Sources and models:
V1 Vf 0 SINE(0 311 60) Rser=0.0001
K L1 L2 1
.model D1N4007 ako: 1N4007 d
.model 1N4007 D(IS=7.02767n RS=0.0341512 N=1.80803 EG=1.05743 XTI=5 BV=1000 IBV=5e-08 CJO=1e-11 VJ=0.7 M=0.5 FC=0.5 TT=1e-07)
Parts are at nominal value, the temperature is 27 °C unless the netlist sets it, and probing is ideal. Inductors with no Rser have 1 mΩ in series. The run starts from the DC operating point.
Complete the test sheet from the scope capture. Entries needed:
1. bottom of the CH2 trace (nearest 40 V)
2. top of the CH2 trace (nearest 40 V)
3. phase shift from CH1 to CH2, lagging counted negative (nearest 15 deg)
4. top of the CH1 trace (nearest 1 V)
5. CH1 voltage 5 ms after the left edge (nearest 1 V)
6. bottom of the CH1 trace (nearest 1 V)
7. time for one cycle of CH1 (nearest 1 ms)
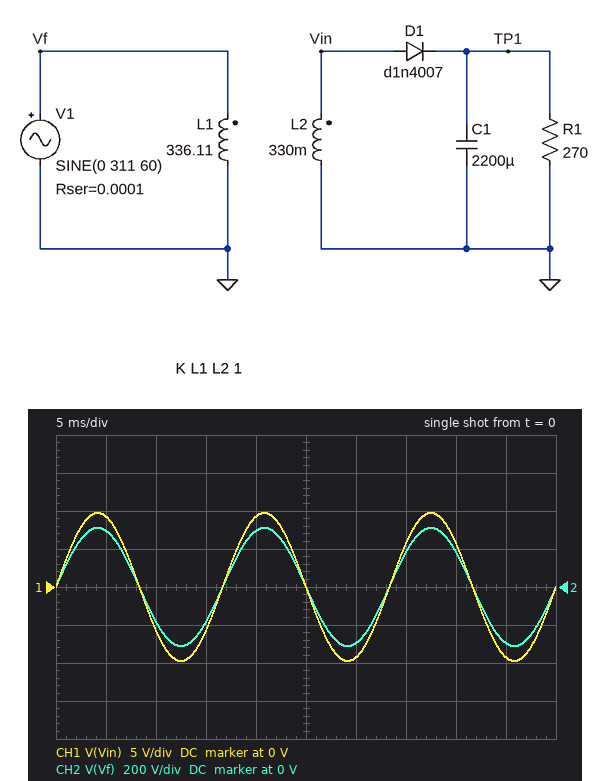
-320 V
320 V
0 deg
10 V
9 V
-10 V
17 ms
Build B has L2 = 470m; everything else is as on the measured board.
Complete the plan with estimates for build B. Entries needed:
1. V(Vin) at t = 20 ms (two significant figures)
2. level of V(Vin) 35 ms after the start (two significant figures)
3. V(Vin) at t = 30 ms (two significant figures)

11 V
6.8 V
-11 V
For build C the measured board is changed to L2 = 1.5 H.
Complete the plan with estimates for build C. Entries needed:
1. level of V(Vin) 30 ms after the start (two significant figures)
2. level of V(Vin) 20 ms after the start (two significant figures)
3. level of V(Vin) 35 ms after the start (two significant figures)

-20 V
20 V
12 V
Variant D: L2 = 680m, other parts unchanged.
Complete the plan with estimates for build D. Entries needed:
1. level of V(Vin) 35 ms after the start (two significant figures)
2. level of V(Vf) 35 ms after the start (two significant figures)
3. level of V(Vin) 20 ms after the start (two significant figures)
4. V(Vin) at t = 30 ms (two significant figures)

8.2 V
180 V
13 V
-13 V
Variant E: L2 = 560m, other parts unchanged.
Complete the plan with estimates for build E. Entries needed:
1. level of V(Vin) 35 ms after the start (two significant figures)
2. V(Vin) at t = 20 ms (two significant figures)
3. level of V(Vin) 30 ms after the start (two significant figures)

7.5 V
12 V
-12 V
